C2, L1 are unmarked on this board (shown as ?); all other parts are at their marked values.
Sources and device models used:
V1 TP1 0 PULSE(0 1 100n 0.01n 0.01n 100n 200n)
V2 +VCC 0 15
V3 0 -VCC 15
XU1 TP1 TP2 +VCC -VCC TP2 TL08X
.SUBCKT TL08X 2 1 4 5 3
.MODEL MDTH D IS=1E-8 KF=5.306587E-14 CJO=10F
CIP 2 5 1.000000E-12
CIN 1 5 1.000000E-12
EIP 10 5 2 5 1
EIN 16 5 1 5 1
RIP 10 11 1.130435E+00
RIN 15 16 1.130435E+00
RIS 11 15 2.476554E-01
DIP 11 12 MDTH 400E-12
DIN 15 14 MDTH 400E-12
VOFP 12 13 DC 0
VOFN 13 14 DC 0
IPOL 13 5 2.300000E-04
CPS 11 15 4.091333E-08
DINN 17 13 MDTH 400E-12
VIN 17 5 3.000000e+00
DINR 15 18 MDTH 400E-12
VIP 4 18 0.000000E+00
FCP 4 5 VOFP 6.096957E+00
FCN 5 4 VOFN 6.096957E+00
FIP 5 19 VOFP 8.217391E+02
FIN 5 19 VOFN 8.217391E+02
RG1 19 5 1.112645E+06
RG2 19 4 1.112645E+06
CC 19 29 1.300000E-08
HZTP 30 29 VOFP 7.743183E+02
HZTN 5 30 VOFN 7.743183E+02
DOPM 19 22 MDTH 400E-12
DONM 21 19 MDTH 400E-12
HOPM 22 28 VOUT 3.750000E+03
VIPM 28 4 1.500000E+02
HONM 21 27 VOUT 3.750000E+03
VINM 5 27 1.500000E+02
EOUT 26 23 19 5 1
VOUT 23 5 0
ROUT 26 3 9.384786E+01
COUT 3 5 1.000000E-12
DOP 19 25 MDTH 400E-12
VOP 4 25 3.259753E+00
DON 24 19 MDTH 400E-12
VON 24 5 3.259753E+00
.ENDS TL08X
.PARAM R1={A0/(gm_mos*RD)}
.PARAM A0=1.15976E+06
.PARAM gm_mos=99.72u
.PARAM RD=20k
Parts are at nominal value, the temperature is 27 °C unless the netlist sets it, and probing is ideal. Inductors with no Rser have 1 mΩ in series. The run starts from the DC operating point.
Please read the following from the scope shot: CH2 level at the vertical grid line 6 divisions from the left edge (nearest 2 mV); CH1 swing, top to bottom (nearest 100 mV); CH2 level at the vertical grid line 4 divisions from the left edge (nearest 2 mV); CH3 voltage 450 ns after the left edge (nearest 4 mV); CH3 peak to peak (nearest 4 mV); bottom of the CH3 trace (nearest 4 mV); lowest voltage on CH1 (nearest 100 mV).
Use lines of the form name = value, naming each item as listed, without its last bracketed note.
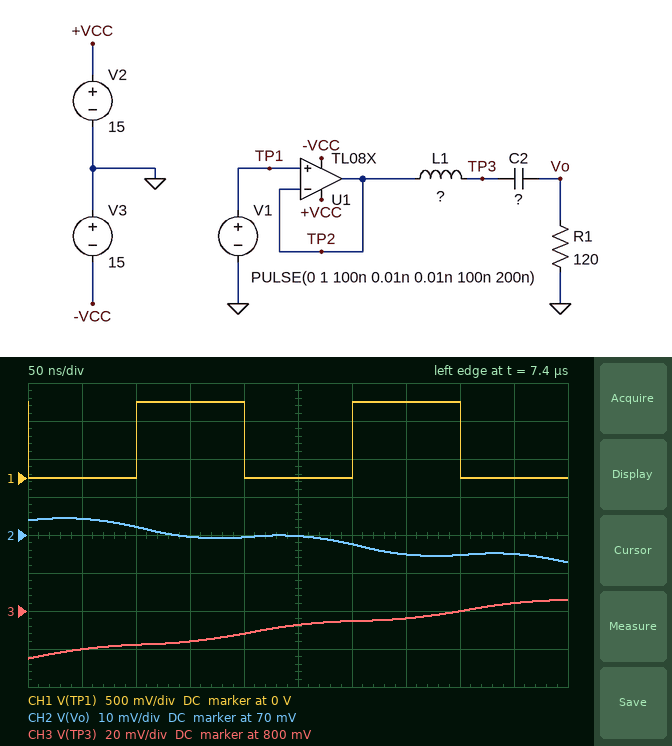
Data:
CH2 level at the vertical grid line 6 divisions from the left edge = 68 mV
CH1 swing, top to bottom = 1.0 V
CH2 level at the vertical grid line 4 divisions from the left edge = 70 mV
CH3 voltage 450 ns after the left edge = 804 mV
CH3 peak to peak = 32 mV
bottom of the CH3 trace = 776 mV
lowest voltage on CH1 = 0 V
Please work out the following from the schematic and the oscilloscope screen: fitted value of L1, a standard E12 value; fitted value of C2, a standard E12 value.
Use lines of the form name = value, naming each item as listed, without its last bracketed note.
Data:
fitted value of L1, a standard E12 value = 1.5 mH
fitted value of C2, a standard E12 value = 6.8 nF
